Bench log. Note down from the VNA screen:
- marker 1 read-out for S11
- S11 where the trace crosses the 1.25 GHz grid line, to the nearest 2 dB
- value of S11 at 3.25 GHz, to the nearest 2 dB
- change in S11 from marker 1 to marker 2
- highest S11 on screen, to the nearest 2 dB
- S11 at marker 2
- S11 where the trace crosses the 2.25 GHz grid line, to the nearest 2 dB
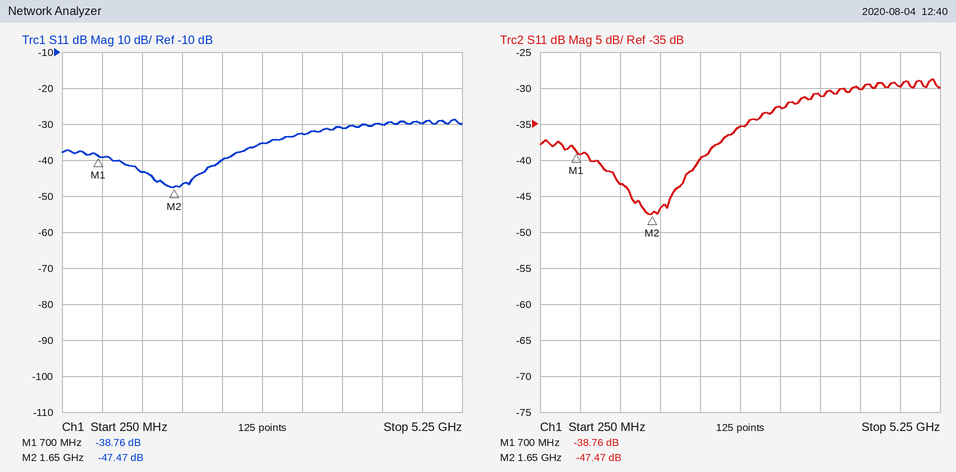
-38.76 dB
-44 dB
-32 dB
-8.71 dB
-28 dB
-47.47 dB
-40 dB
